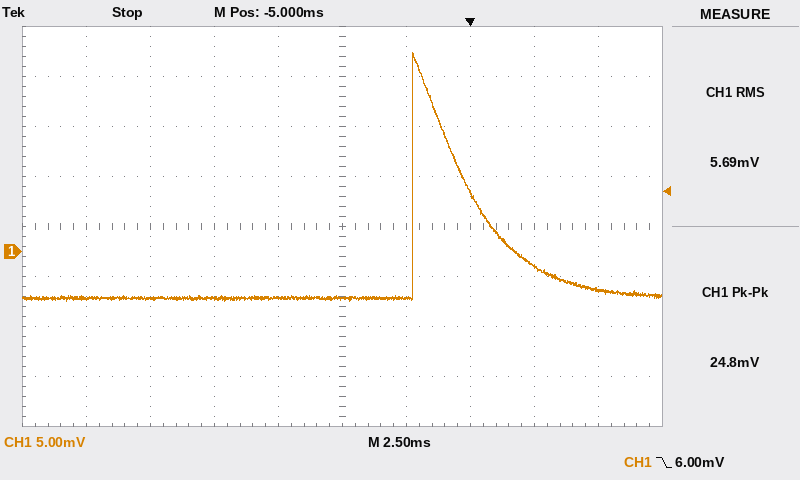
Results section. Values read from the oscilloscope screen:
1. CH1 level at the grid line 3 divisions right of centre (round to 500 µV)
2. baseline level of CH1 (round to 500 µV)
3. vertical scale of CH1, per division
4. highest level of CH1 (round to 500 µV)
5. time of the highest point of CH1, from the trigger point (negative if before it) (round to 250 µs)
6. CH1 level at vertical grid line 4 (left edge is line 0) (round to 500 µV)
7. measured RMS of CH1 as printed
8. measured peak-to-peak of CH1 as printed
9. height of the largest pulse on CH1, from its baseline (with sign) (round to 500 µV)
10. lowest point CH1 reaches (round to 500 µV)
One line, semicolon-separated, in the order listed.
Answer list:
-1.5 mV; -4.5 mV; 5 mV; 20.0 mV; -2.25 ms; -4.5 mV; 5.69 mV; 24.8 mV; +24.5 mV; -5.0 mV
